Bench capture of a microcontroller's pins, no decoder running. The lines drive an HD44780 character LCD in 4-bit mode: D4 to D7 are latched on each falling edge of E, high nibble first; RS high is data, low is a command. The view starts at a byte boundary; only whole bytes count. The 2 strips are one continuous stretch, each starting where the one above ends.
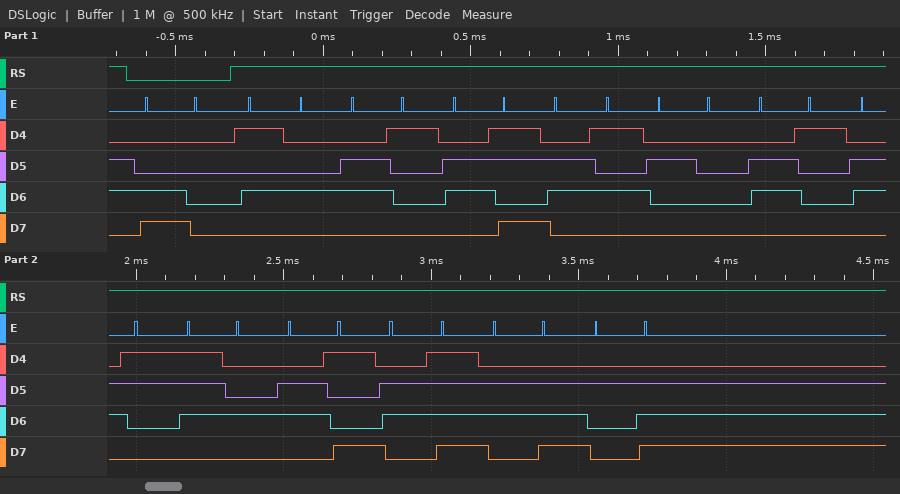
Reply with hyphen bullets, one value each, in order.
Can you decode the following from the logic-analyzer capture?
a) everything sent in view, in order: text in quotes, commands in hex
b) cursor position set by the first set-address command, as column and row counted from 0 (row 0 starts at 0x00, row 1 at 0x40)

- 0xC0 "Take action."
- column 0, row 1
